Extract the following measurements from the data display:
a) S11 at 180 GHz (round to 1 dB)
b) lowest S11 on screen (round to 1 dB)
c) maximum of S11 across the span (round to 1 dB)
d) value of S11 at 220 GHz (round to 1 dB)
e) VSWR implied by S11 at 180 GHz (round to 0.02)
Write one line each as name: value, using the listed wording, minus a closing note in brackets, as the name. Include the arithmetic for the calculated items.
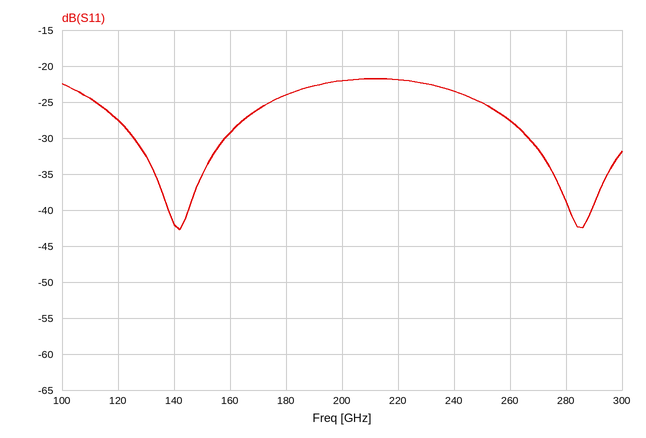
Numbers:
S11 at 180 GHz: -24 dB
lowest S11 on screen: -43 dB
maximum of S11 across the span: -22 dB
value of S11 at 220 GHz: -22 dB
VSWR implied by S11 at 180 GHz: |Γ| = 10^(-24/20) = 0.0631; VSWR = (1 + 0.0631)/(1 − 0.0631) ≈ 1.13, so 1.14 to the nearest 0.02
